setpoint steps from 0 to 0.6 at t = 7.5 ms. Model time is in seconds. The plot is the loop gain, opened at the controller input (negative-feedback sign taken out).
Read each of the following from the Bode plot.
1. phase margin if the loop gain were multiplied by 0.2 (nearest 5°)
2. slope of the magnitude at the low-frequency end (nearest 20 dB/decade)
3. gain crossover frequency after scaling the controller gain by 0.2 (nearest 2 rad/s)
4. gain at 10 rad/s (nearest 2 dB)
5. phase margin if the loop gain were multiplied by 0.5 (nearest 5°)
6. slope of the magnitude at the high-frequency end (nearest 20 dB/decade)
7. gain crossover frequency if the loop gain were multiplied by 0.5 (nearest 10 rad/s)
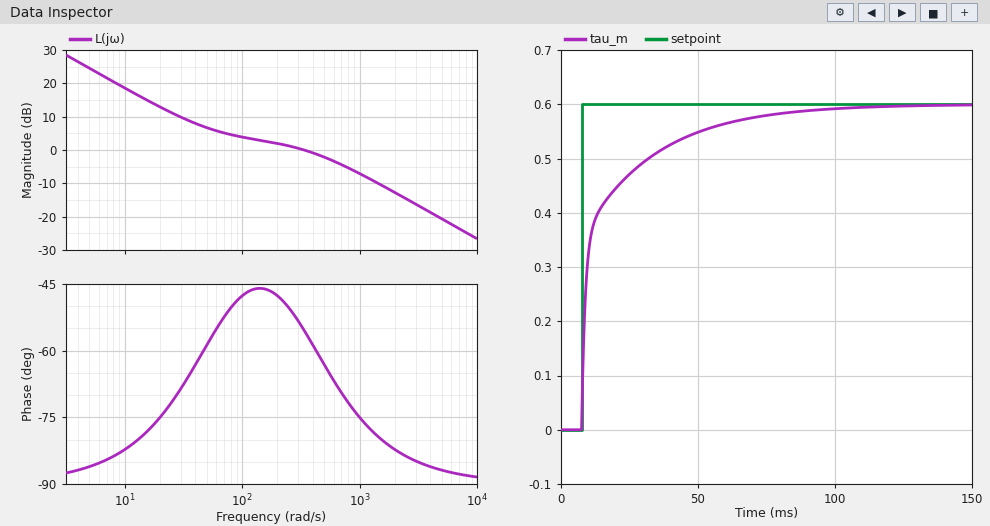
105°
-20 dB/decade
18 rad/s
18 dB
125°
-20 dB/decade
60 rad/s
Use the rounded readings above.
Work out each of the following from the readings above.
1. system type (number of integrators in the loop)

1
